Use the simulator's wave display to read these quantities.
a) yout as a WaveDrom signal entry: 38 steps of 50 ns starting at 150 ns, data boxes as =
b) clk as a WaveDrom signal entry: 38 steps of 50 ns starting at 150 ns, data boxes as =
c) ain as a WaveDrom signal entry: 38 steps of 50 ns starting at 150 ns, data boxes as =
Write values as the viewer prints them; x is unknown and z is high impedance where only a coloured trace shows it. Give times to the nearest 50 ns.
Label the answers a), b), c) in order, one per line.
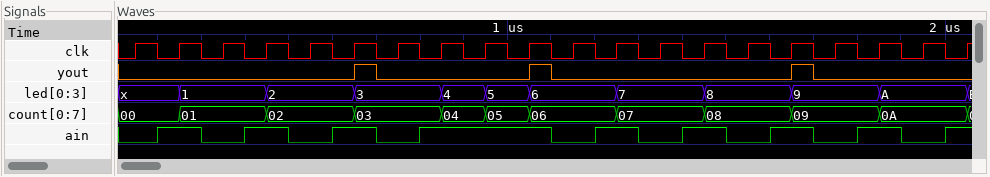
a) {name: 'yout', wave: '0.........10......10..........10......'}
b) {name: 'clk', wave: '10101010101010101010101010101010101010'}
c) {name: 'ain', wave: '01.0.1.0.1.0.1.....0.1.0.1.0.1.0.1.0.1'}
